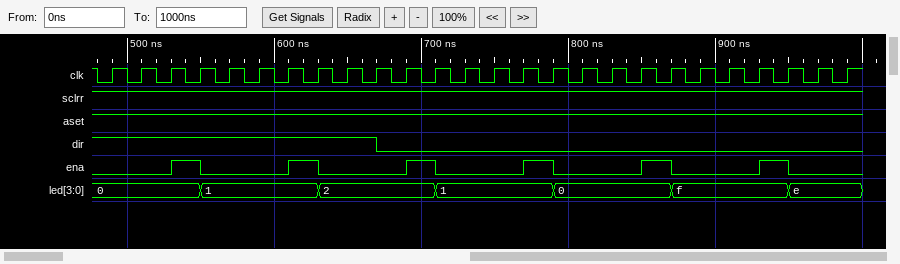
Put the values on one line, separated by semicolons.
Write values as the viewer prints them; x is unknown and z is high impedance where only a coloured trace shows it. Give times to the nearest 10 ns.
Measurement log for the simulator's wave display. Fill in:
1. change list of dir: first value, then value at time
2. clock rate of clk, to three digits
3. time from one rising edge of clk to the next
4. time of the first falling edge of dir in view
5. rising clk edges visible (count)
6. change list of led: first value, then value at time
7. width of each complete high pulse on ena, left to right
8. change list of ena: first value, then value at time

1, 0 at 670 ns; 50.0 MHz; 20 ns; 670 ns; 26; 0, 1 at 550 ns, 2 at 630 ns, 1 at 710 ns, 0 at 790 ns, f at 870 ns, e at 950 ns; 20 ns, 20 ns, 20 ns, 20 ns, 20 ns, 20 ns; 0, 1 at 530 ns, 0 at 550 ns, 1 at 610 ns, 0 at 630 ns, 1 at 690 ns, 0 at 710 ns, 1 at 770 ns, 0 at 790 ns, 1 at 850 ns, 0 at 870 ns, 1 at 930 ns, 0 at 950 ns
